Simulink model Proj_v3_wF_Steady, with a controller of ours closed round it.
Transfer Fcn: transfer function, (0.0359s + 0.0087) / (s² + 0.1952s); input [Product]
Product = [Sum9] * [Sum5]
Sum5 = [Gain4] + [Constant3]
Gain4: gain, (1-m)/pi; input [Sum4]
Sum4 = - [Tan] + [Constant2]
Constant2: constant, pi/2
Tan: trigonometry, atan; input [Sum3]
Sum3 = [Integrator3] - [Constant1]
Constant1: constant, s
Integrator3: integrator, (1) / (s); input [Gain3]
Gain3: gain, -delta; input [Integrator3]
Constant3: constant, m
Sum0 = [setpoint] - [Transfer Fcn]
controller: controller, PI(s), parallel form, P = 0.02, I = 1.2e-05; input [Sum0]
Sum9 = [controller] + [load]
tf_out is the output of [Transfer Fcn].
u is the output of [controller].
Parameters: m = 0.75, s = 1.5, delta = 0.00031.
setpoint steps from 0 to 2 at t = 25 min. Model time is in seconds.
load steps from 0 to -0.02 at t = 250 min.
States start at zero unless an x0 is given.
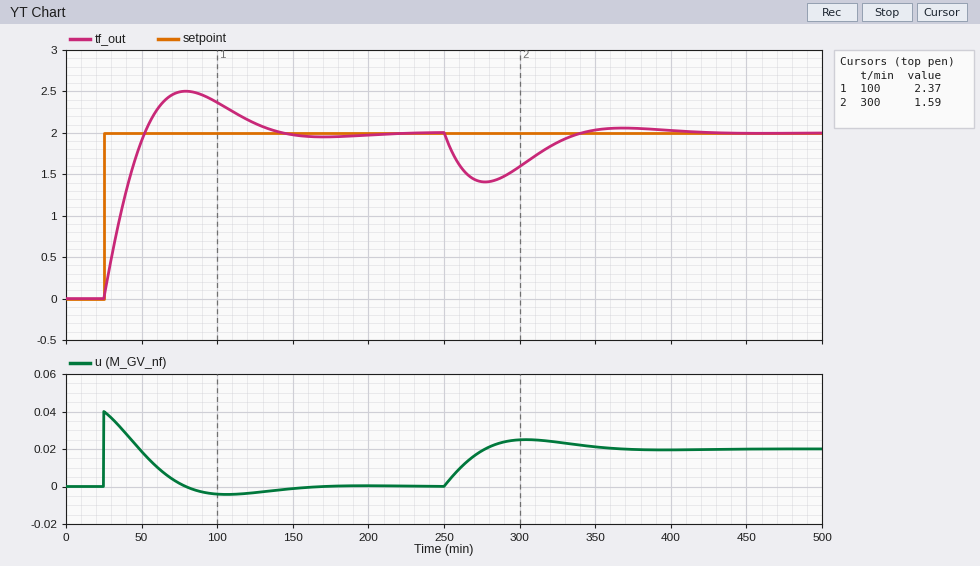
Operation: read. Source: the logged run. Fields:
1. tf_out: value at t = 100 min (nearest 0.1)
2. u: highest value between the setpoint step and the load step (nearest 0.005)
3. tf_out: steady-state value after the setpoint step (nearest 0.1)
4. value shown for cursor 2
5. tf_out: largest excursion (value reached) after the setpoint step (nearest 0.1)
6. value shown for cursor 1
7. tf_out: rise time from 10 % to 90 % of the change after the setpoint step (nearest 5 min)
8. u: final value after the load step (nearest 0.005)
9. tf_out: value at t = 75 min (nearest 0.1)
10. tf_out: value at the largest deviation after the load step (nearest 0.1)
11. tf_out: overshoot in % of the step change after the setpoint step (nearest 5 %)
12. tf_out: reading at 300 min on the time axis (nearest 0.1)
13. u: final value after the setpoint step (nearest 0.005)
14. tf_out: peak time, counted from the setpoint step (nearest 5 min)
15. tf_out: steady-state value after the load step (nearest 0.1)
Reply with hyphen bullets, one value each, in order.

- 2.4
- 0.040
- 2.0
- 1.59
- 2.5
- 2.37
- 20 min
- 0.020
- 2.5
- 1.4
- 25 %
- 1.6
- 0.000
- 55 min
- 2.0
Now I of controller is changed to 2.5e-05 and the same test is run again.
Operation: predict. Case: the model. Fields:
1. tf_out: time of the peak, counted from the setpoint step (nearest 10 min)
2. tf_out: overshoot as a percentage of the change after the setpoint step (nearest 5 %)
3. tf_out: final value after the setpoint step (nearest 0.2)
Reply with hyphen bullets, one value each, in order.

- 40 min
- 35 %
- 2.0
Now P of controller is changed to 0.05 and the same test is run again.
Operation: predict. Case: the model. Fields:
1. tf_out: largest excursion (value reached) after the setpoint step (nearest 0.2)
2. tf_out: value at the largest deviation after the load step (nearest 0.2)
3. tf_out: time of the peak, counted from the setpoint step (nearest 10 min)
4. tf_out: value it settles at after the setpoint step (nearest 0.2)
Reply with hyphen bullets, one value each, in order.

- 2.2
- 1.6
- 40 min
- 2.0
